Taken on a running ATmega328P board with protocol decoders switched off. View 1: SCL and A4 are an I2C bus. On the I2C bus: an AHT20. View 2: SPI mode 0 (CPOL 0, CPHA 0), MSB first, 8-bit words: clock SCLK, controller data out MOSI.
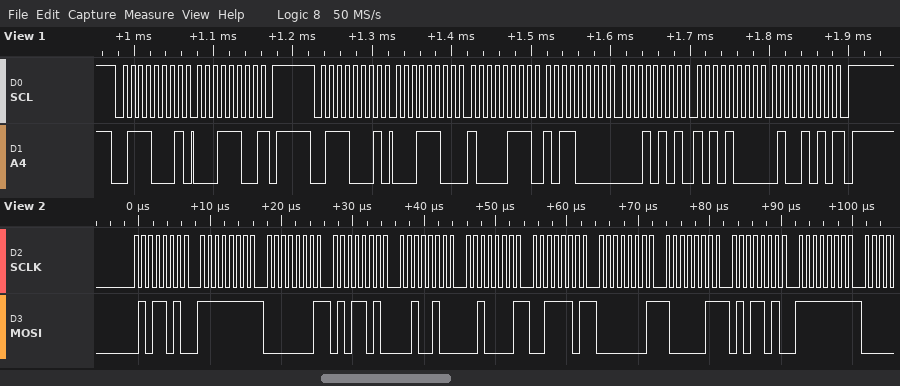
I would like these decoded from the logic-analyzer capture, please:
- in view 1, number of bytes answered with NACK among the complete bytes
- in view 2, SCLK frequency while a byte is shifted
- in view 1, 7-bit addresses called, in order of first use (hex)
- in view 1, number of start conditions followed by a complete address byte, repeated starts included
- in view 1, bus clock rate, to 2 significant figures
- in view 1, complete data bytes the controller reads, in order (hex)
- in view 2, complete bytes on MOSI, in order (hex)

2
1 MHz
0x38
2
100 kHz
1C 1C 87 B0 15 A8 4A
0x5A 0xFF 0x01 0x5A 0x24 0x21 0x3D 0x01 0x83 0x5A 0xFF
